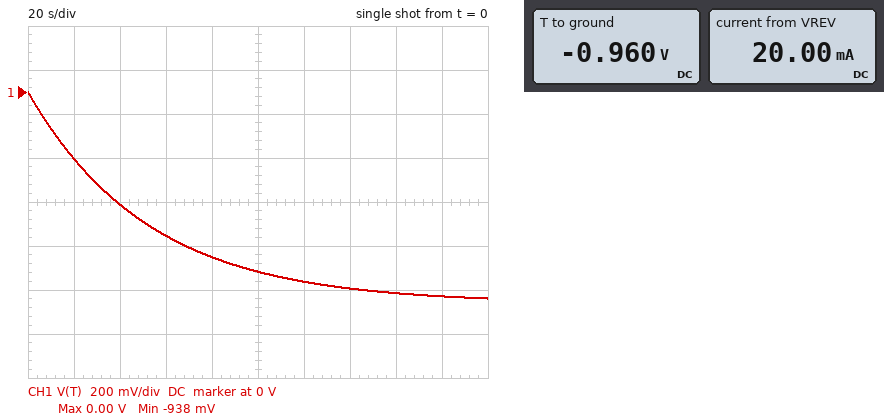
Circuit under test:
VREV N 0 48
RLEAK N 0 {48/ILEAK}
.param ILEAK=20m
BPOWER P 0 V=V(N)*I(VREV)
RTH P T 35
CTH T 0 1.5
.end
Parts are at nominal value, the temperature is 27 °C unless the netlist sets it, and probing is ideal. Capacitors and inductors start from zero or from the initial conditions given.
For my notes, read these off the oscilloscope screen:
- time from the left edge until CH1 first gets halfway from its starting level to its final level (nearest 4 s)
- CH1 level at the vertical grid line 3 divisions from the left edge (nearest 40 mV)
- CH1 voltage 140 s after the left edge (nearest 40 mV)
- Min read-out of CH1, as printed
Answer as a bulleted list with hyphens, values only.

- 36 s
- -640 mV
- -880 mV
- -938 mV
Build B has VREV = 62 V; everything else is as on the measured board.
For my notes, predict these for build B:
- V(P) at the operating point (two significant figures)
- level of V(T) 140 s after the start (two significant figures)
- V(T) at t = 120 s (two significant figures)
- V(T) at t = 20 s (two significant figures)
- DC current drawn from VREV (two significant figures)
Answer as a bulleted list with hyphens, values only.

- -1.6 V
- -1.5 V
- -1.4 V
- -510 mV
- 26 mA
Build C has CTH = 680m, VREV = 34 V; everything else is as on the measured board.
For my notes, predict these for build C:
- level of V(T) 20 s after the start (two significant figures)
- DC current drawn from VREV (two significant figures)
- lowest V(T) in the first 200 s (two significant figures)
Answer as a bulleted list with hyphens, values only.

- -270 mV
- 14 mA
- -480 mV
